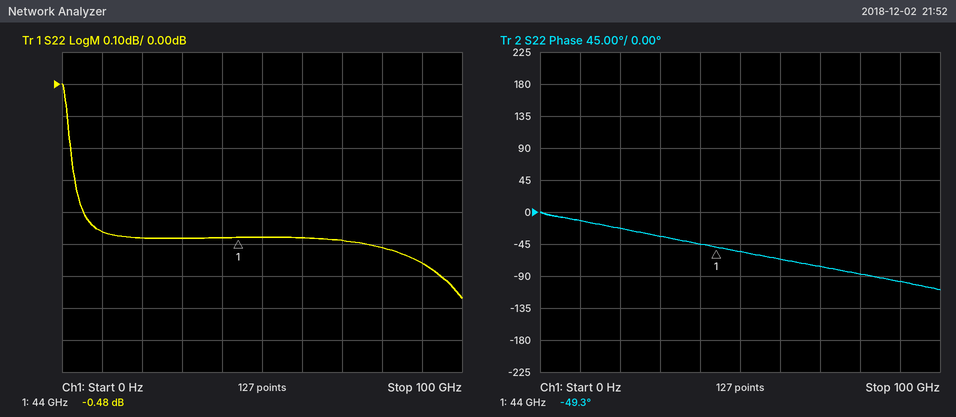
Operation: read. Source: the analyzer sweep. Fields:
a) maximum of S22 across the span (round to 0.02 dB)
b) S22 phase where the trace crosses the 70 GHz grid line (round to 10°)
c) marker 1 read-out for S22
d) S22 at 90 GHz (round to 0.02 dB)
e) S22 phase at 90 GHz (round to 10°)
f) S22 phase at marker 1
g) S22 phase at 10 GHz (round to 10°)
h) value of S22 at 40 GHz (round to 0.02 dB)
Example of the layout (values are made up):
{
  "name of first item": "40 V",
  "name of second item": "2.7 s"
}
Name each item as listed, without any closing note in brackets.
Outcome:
{
  "maximum of S22 across the span": "0.00 dB",
  "S22 phase where the trace crosses the 70 GHz grid line": "-80°",
  "marker 1 read-out for S22": "-0.48 dB",
  "S22 at 90 GHz": "-0.56 dB",
  "S22 phase at 90 GHz": "-100°",
  "S22 phase at marker 1": "-49.3°",
  "S22 phase at 10 GHz": "-10°",
  "value of S22 at 40 GHz": "-0.48 dB"
}
